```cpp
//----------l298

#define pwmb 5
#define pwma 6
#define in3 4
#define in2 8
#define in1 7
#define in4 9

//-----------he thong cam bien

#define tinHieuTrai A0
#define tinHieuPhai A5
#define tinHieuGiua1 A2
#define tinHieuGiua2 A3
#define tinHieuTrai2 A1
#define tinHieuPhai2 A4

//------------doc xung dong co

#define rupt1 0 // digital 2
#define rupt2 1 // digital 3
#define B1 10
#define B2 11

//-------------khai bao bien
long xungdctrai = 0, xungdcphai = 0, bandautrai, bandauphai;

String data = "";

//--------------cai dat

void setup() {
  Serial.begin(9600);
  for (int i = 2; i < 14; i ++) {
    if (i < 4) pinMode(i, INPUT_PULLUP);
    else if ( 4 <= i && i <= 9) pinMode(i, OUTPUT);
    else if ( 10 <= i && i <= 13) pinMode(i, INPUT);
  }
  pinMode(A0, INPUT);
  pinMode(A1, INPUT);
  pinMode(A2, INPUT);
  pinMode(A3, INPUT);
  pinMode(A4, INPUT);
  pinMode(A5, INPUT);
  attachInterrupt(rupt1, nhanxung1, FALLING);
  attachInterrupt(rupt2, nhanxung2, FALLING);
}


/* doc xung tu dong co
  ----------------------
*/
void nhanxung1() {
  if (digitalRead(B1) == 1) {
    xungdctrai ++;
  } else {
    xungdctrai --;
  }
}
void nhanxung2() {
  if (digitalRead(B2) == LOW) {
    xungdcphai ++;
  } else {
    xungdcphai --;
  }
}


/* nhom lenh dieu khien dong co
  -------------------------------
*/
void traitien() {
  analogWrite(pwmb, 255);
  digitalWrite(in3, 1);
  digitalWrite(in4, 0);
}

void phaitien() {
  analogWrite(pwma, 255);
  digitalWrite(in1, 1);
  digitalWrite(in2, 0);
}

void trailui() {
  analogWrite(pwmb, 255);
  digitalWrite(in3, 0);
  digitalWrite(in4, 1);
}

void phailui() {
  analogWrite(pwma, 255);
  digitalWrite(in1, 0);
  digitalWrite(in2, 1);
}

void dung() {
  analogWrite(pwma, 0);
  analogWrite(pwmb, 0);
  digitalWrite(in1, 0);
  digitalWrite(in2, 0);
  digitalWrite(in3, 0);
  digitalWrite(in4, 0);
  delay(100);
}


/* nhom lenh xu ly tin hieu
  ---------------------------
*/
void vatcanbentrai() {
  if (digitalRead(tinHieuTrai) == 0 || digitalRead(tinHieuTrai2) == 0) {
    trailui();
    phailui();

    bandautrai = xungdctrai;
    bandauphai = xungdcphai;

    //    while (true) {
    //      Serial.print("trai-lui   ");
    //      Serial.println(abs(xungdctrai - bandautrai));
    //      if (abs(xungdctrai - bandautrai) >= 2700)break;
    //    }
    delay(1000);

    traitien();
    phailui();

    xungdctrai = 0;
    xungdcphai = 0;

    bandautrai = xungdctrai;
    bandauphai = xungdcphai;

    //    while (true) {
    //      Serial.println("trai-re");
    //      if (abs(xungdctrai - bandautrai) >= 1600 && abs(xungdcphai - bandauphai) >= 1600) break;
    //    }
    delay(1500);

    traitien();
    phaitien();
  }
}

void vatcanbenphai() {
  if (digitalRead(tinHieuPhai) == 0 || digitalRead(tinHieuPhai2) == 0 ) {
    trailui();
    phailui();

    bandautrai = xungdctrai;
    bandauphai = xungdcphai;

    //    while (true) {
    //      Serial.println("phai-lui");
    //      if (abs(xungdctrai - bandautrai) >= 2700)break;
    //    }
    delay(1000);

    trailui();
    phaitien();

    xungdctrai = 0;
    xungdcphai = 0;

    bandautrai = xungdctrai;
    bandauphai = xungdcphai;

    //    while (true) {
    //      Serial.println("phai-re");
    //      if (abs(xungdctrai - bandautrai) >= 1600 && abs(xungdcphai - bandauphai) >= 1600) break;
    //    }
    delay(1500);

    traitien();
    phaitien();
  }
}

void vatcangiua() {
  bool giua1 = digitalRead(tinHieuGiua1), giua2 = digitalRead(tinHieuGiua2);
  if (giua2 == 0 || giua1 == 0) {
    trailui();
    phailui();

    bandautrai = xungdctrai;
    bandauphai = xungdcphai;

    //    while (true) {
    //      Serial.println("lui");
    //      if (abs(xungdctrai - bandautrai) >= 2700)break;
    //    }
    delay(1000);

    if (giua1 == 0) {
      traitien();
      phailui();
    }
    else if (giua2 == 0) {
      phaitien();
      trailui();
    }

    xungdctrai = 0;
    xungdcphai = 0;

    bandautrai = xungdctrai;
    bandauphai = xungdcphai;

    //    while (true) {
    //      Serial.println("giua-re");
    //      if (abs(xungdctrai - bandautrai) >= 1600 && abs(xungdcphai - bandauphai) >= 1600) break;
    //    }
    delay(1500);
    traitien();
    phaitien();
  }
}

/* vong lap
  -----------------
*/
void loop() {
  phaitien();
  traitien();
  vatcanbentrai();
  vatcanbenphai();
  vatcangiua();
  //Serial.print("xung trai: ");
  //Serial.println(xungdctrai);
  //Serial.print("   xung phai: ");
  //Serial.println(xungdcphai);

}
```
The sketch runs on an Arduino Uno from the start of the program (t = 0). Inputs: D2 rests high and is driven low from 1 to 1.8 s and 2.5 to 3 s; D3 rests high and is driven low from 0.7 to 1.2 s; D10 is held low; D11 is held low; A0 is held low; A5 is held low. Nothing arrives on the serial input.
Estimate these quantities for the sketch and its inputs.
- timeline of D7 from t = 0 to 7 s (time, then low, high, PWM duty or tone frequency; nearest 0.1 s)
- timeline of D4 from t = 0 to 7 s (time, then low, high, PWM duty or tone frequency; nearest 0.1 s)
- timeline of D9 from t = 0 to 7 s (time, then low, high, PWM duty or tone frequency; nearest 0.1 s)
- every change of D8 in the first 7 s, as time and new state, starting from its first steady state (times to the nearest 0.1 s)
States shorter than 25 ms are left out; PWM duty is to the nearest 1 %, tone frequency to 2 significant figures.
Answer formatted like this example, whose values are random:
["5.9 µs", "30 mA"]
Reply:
["0 s low; 3.5 s high; 5 s low", "0 s low; 1 s high; 2.5 s low; 6 s high", "0 s high; 1 s low; 2.5 s high; 6 s low", "0 s high; 3.5 s low; 5 s high"]
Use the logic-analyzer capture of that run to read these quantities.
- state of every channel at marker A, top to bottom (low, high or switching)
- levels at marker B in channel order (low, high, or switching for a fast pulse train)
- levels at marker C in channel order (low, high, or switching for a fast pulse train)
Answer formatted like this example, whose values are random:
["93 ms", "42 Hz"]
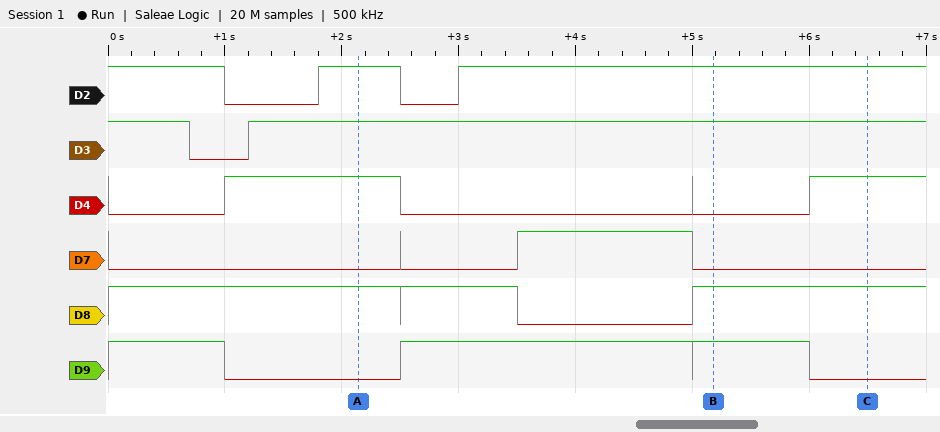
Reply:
["D2 high, D3 high, D4 high, D7 low, D8 high, D9 low", "D2 high, D3 high, D4 low, D7 low, D8 high, D9 high", "D2 high, D3 high, D4 high, D7 low, D8 high, D9 low"]
